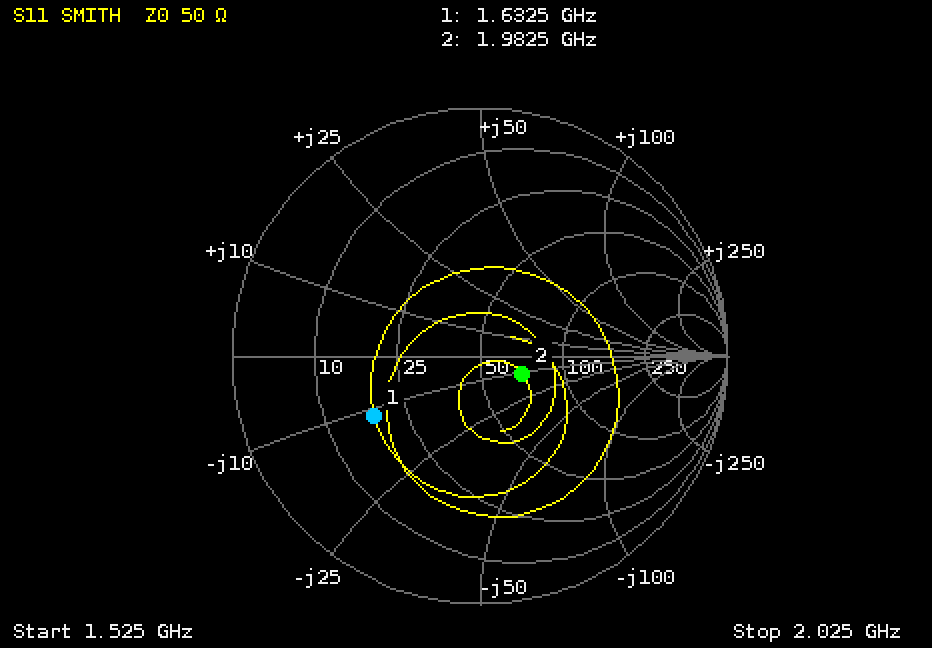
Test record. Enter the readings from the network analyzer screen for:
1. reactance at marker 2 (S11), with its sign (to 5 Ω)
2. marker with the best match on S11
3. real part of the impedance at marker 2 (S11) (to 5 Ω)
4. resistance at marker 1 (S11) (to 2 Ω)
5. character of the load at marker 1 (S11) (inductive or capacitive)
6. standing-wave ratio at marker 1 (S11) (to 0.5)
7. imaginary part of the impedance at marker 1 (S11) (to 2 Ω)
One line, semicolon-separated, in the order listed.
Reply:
-10 Ω; marker 2; 70 Ω; 18 Ω; capacitive; 3.0; -12 Ω
